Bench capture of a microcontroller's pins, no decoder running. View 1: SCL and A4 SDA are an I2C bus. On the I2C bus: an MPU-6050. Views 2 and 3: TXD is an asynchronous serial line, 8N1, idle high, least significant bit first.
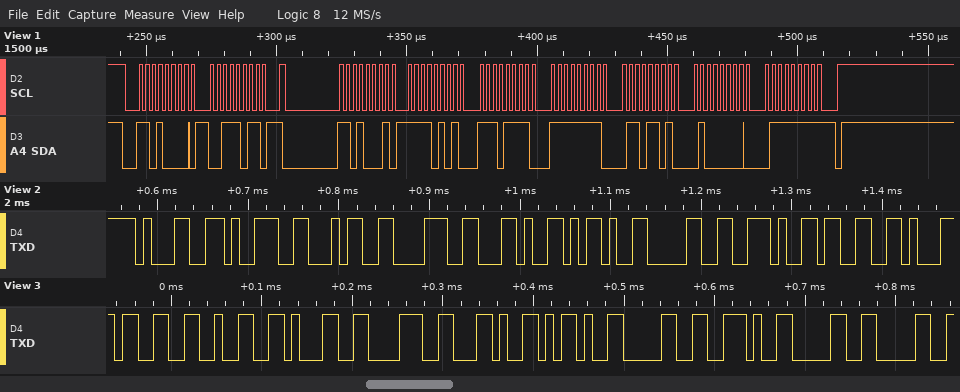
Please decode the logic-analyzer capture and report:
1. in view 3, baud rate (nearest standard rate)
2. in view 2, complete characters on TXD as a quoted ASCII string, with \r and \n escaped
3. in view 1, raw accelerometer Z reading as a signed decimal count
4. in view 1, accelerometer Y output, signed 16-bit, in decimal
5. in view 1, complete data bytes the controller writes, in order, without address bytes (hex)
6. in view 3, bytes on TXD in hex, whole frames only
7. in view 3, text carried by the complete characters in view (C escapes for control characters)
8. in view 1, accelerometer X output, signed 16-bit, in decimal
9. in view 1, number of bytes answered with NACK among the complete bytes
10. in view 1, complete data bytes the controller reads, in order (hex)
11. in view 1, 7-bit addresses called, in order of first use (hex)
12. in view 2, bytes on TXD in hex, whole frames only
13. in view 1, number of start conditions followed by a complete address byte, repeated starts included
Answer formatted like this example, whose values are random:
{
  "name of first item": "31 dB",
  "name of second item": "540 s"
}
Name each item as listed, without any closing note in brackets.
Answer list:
{
  "in view 3, baud rate": "115200 baud",
  "in view 2, complete characters on TXD as a quoted ASCII string, with \\r and \\n escaped": "\"1948,-0.3\"",
  "in view 1, raw accelerometer Z reading as a signed decimal count": "16511",
  "in view 1, accelerometer Y output, signed 16-bit, in decimal": "-147",
  "in view 1, complete data bytes the controller writes, in order, without address bytes": "3B",
  "in view 3, bytes on TXD in hex, whole frames only": "0x33 0x32 0x31 0x38 0x2C 0x2D 0x30 0x2E 0x30 0x30",
  "in view 3, text carried by the complete characters in view": "\"3218,-0.00\"",
  "in view 1, accelerometer X output, signed 16-bit, in decimal": "-2577",
  "in view 1, number of bytes answered with NACK among the complete bytes": "1",
  "in view 1, complete data bytes the controller reads, in order": "F5 EF FF 6D 40 7F",
  "in view 1, 7-bit addresses called, in order of first use": "0x68",
  "in view 2, bytes on TXD in hex, whole frames only": "0x31 0x39 0x34 0x38 0x2C 0x2D 0x30 0x2E 0x33",
  "in view 1, number of start conditions followed by a complete address byte, repeated starts included": "2"
}
